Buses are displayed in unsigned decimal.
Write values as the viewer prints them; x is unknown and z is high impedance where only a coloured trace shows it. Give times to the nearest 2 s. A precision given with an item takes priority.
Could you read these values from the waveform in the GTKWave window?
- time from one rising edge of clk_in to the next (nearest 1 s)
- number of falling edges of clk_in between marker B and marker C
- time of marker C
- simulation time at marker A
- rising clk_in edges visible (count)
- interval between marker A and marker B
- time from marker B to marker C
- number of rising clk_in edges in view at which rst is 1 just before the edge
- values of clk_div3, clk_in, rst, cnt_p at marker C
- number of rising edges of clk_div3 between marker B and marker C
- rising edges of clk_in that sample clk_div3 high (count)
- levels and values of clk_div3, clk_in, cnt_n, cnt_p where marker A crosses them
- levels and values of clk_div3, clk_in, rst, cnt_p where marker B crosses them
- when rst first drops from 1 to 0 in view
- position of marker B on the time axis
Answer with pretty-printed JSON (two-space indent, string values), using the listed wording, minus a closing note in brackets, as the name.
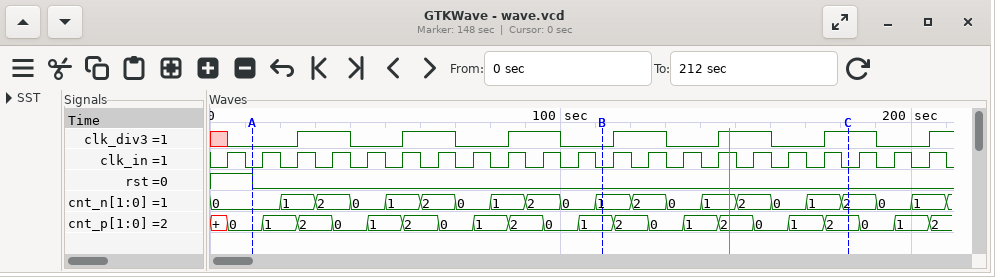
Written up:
{
  "time from one rising edge of clk_in to the next": "10 s",
  "number of falling edges of clk_in between marker B and marker C": "7",
  "time of marker C": "182 s",
  "simulation time at marker A": "12 s",
  "rising clk_in edges visible": "21",
  "interval between marker A and marker B": "100 s",
  "time from marker B to marker C": "70 s",
  "number of rising clk_in edges in view at which rst is 1 just before the edge": "1",
  "values of clk_div3, clk_in, rst, cnt_p at marker C": "clk_div3=1, clk_in=0, rst=0, cnt_p=2",
  "number of rising edges of clk_div3 between marker B and marker C": "3",
  "rising edges of clk_in that sample clk_div3 high": "6",
  "levels and values of clk_div3, clk_in, cnt_n, cnt_p where marker A crosses them": "clk_div3=0, clk_in=0, cnt_n=0, cnt_p=0",
  "levels and values of clk_div3, clk_in, rst, cnt_p where marker B crosses them": "clk_div3=0, clk_in=0, rst=0, cnt_p=1",
  "when rst first drops from 1 to 0 in view": "12 s",
  "position of marker B on the time axis": "112 s"
}
